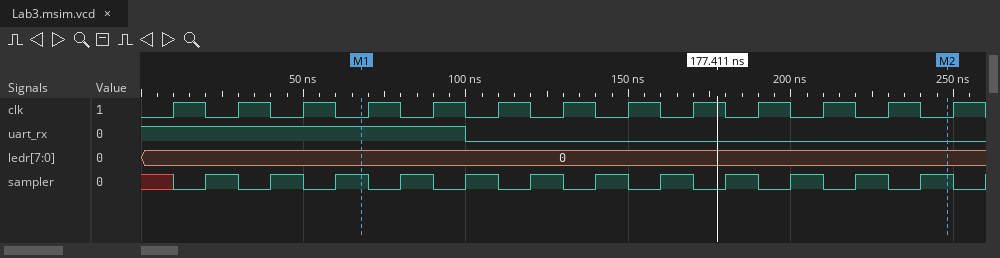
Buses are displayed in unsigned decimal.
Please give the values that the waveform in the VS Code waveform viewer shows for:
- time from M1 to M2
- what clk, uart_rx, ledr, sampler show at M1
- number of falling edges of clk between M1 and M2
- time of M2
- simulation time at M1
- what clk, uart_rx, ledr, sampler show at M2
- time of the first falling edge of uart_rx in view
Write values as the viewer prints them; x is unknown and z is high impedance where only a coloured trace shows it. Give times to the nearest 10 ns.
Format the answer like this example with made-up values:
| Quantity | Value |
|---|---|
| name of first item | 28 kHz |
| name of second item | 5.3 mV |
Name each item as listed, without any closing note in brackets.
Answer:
| Quantity | Value |
|---|---|
| time from M1 to M2 | 180 ns |
| what clk, uart_rx, ledr, sampler show at M1 | clk=0, uart_rx=1, ledr=0, sampler=1 |
| number of falling edges of clk between M1 and M2 | 9 |
| time of M2 | 250 ns |
| simulation time at M1 | 70 ns |
| what clk, uart_rx, ledr, sampler show at M2 | clk=0, uart_rx=0, ledr=0, sampler=1 |
| time of the first falling edge of uart_rx in view | 100 ns |
